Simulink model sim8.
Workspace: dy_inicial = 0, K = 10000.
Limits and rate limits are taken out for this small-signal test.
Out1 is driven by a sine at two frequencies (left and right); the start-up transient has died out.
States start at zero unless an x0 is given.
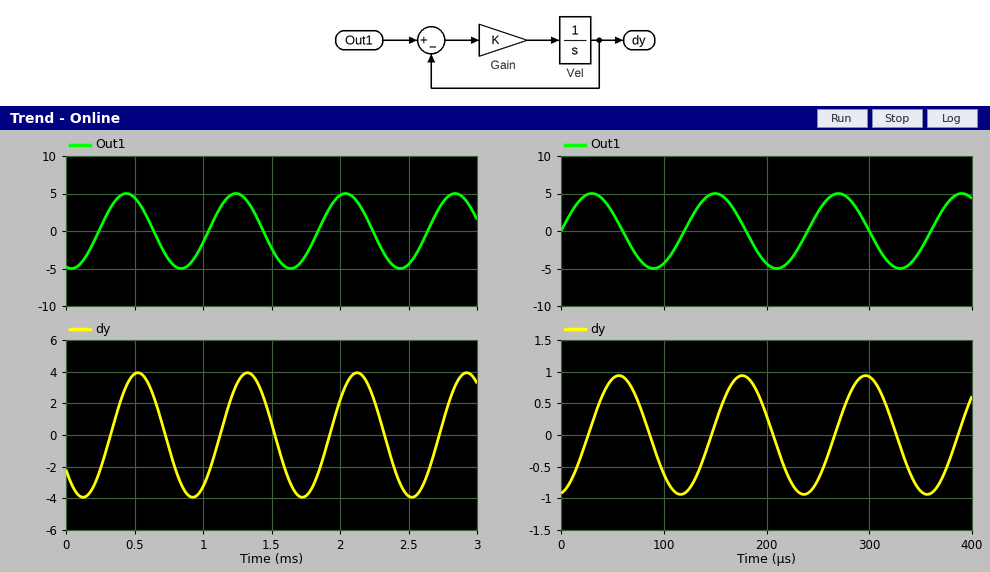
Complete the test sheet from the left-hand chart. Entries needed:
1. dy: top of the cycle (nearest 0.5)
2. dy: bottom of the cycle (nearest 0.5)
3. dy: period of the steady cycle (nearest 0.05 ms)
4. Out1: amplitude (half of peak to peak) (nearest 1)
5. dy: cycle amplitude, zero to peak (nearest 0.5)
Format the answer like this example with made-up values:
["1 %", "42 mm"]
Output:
["4.0", "-4.0", "0.80 ms", "5", "4.0"]
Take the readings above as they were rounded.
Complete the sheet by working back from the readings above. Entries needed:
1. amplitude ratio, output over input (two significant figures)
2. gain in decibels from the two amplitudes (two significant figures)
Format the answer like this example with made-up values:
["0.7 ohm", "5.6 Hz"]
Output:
["0.80", "-1.9 dB"]
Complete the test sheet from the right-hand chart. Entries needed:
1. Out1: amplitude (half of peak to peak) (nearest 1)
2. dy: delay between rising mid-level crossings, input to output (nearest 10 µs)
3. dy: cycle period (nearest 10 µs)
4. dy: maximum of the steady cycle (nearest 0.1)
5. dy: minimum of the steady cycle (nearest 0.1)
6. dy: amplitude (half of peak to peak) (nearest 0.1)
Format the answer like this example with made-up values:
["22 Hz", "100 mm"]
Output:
["5", "30 µs", "120 µs", "0.9", "-0.9", "0.9"]
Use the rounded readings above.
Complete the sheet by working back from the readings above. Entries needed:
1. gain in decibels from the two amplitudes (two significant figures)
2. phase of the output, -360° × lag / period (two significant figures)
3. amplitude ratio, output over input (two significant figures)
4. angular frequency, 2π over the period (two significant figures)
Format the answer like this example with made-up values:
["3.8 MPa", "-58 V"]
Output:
["-15 dB", "-90°", "0.18", "0.052 rad/µs"]
